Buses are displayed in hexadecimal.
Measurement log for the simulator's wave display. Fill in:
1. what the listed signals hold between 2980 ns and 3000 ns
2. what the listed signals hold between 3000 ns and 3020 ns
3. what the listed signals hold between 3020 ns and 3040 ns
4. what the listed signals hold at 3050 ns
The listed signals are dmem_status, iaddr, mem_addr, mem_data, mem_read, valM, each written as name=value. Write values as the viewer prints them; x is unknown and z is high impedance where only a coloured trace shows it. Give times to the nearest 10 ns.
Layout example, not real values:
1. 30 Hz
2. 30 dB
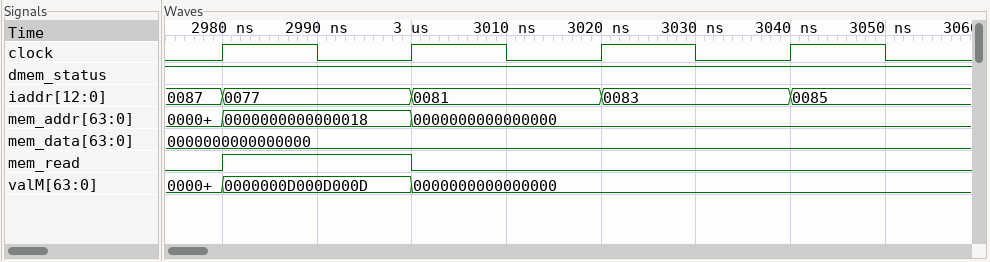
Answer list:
1. dmem_status=1, iaddr=0077, mem_addr=0000000000000018, mem_data=0000000000000000, mem_read=1, valM=0000000D000D000D
2. dmem_status=1, iaddr=0081, mem_addr=0000000000000000, mem_data=0000000000000000, mem_read=0, valM=0000000000000000
3. dmem_status=1, iaddr=0083, mem_addr=0000000000000000, mem_data=0000000000000000, mem_read=0, valM=0000000000000000
4. dmem_status=1, iaddr=0085, mem_addr=0000000000000000, mem_data=0000000000000000, mem_read=0, valM=0000000000000000
